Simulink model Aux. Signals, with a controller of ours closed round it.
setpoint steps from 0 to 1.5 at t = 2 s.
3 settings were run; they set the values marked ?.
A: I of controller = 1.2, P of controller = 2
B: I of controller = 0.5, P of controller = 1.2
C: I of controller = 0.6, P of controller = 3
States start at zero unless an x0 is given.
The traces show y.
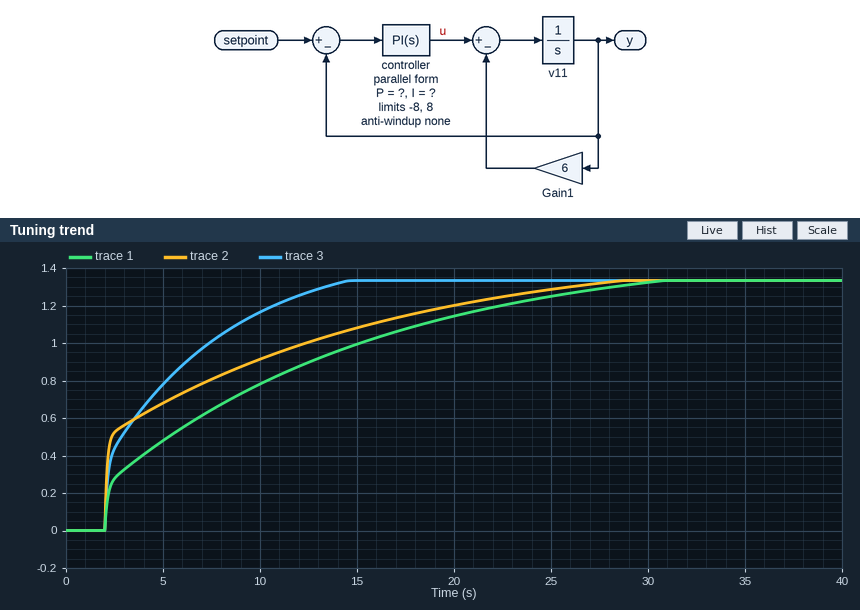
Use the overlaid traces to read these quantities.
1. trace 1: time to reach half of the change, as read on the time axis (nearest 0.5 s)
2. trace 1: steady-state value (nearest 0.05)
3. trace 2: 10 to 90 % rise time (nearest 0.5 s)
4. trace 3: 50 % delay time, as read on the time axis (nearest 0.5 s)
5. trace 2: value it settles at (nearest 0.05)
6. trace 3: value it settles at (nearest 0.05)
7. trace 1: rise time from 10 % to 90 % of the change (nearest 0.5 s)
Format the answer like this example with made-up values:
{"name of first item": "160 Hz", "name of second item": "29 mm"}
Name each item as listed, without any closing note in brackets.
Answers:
{"trace 1: time to reach half of the change, as read on the time axis": "8.0 s", "trace 1: steady-state value": "1.35", "trace 2: 10 to 90 % rise time": "18.0 s", "trace 3: 50 % delay time, as read on the time axis": "4.0 s", "trace 2: value it settles at": "1.35", "trace 3: value it settles at": "1.35", "trace 1: rise time from 10 % to 90 % of the change": "20.5 s"}
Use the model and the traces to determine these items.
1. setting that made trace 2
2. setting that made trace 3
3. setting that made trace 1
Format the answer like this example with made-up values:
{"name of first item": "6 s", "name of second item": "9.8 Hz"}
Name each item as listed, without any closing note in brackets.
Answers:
{"setting that made trace 2": "C", "setting that made trace 3": "A", "setting that made trace 1": "B"}
